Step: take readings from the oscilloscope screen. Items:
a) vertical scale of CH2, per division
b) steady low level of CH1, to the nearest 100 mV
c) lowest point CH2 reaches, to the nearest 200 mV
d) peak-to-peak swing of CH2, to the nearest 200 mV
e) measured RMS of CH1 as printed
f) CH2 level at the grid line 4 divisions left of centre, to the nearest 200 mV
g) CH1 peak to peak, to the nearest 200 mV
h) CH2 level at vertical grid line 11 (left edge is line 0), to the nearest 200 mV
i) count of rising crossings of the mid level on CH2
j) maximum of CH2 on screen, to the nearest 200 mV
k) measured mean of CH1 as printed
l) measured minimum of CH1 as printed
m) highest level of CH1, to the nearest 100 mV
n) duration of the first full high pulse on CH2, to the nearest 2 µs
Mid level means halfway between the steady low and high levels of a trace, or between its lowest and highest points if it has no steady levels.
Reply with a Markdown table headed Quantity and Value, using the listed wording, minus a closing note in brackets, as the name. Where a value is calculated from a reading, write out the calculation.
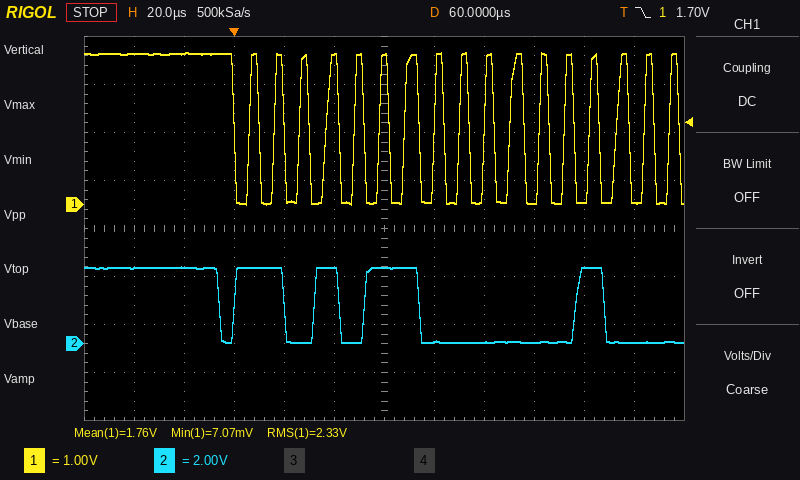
| Quantity | Value |
|---|---|
| vertical scale of CH2, per division | 2 V |
| steady low level of CH1, to the nearest 100 mV | 0.0 V |
| lowest point CH2 reaches, to the nearest 200 mV | 0.0 V |
| peak-to-peak swing of CH2, to the nearest 200 mV | 3.2 V − (0.0 V) = 3.2 V |
| measured RMS of CH1 as printed | 2.33 V |
| CH2 level at the grid line 4 divisions left of centre, to the nearest 200 mV | 3.2 V |
| CH1 peak to peak, to the nearest 200 mV | 3.2 V |
| CH2 level at vertical grid line 11 (left edge is line 0), to the nearest 200 mV | 0.0 V |
| count of rising crossings of the mid level on CH2 | 4 |
| maximum of CH2 on screen, to the nearest 200 mV | 3.2 V |
| measured mean of CH1 as printed | 1.76 V |
| measured minimum of CH1 as printed | 7.07 mV |
| highest level of CH1, to the nearest 100 mV | 3.2 V |
| duration of the first full high pulse on CH2, to the nearest 2 µs | 20 µs |
